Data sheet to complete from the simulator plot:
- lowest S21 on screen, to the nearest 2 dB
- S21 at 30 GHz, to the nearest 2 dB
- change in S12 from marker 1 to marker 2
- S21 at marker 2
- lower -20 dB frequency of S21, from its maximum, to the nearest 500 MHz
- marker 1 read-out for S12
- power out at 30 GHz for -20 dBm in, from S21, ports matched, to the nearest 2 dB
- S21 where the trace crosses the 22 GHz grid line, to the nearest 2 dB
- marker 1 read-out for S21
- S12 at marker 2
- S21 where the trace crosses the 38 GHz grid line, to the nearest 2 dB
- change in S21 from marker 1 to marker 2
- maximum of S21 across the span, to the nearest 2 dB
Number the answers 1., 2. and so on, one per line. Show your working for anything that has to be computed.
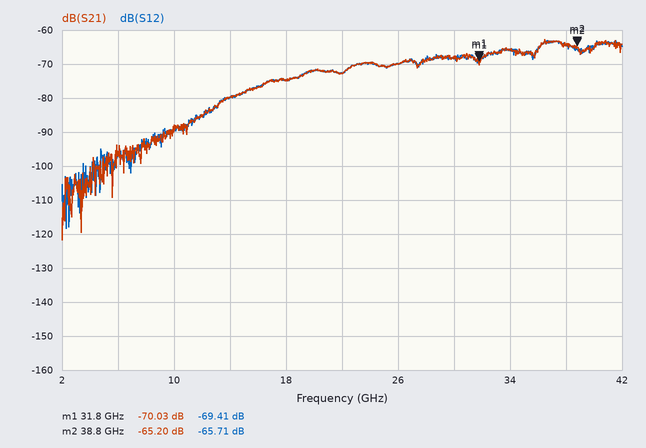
1. -122 dB
2. -68 dB
3. -65.71 − (-69.41) = 3.70 dB
4. -65.20 dB
5. 13.0 GHz
6. -69.41 dB
7. -20 dBm + (-68 dB) = -88 dBm
8. -72 dB
9. -70.03 dB
10. -65.71 dB
11. -64 dB
12. -65.2 − (-70.03) = 4.83 dB
13. -62 dB
